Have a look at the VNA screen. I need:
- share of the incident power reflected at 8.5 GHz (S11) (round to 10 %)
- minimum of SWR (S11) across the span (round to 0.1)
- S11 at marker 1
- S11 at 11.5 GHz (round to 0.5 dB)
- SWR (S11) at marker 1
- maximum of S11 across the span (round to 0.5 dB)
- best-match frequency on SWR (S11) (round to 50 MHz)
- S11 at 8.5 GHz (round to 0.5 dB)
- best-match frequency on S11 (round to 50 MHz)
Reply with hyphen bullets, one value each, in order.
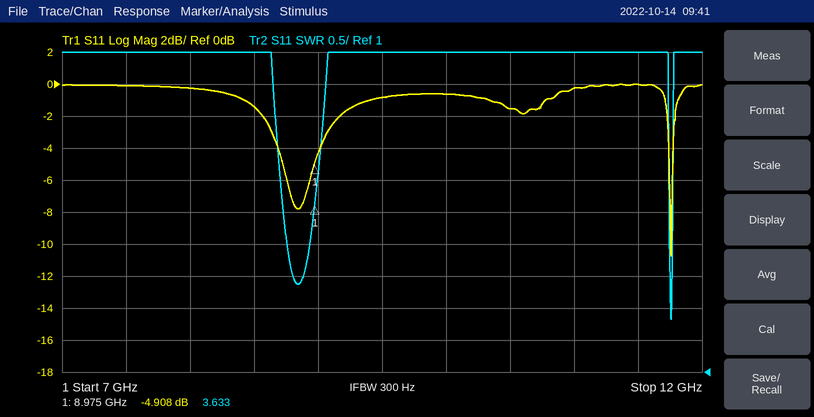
- 70 %
- 1.8
- -4.908 dB
- 0.0 dB
- 3.633
- 0.0 dB
- 11.75 GHz
- -1.5 dB
- 11.75 GHz
